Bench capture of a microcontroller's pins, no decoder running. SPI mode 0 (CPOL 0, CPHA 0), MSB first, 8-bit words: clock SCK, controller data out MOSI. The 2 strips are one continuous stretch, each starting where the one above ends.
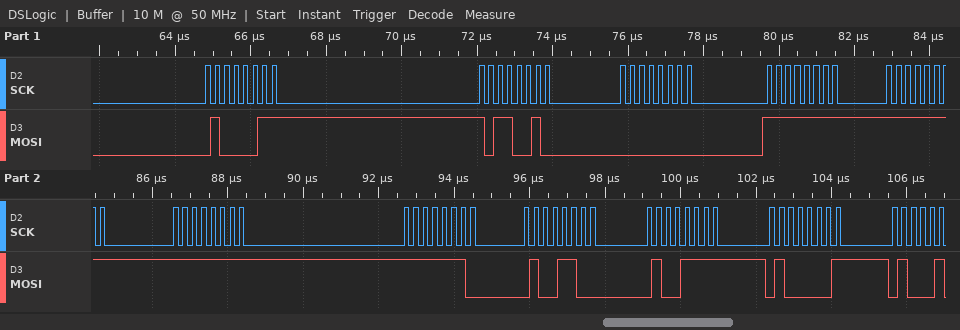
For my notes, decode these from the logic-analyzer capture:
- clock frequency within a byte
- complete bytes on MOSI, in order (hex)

4 MHz
0x43 0xB2 0x00 0xFF 0xFF 0xFF 0xFE 0x4C 0x4F 0x41
